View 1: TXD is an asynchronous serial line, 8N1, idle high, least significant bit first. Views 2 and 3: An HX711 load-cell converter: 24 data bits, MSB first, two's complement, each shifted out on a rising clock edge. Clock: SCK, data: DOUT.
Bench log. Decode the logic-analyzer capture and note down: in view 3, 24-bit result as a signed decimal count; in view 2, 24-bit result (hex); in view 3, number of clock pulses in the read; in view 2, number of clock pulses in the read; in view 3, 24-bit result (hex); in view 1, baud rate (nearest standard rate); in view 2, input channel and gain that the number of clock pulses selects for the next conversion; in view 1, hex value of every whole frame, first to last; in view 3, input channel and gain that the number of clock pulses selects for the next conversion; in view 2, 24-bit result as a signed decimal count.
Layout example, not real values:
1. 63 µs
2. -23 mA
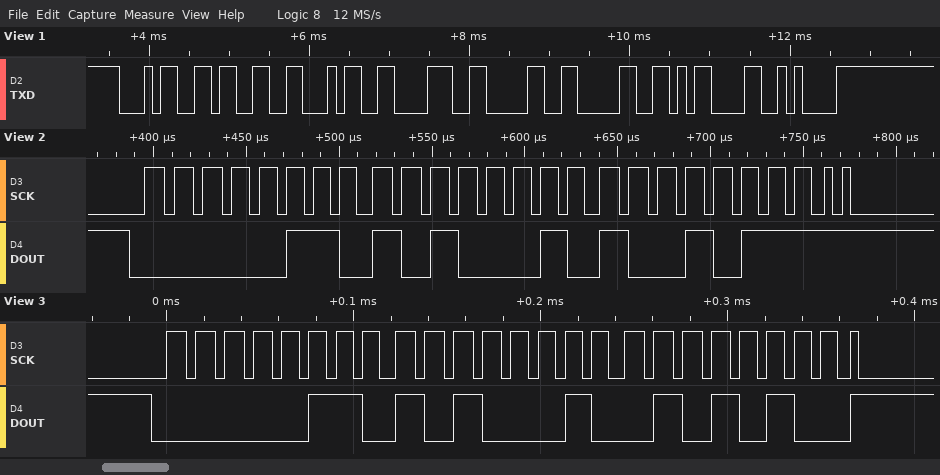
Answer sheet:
1. 434772
2. 0x06A297
3. 25
4. 26
5. 0x06A254
6. 9600 baud
7. channel B, gain 32
8. 34 33 34 38 30 30 0D 0A
9. channel A, gain 128
10. 434839
